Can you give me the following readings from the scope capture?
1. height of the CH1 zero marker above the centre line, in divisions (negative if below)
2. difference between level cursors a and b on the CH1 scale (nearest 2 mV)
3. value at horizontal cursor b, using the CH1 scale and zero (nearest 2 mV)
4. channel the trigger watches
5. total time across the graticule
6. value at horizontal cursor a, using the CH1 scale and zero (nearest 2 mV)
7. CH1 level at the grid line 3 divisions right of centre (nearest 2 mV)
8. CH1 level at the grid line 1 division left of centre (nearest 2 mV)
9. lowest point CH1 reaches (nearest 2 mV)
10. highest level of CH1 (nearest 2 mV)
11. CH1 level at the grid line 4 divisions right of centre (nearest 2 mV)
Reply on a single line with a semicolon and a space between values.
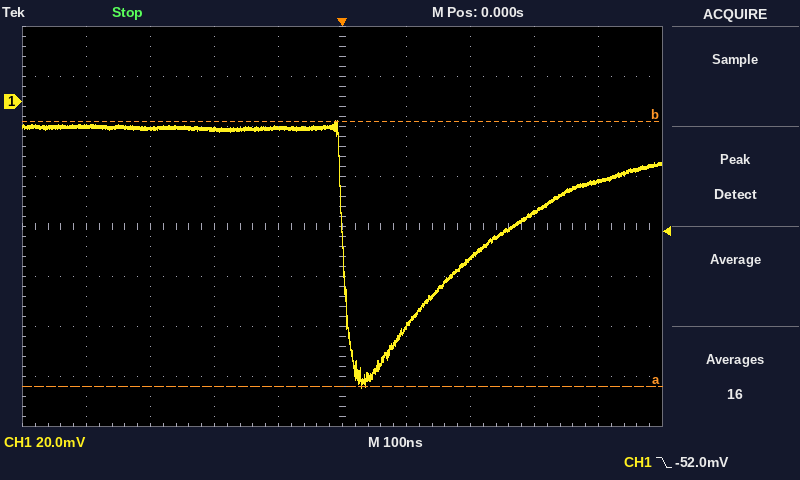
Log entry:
+2.5 div; 106 mV; -8 mV; CH1; 1 µs; -114 mV; -44 mV; -10 mV; -114 mV; -8 mV; -32 mV
